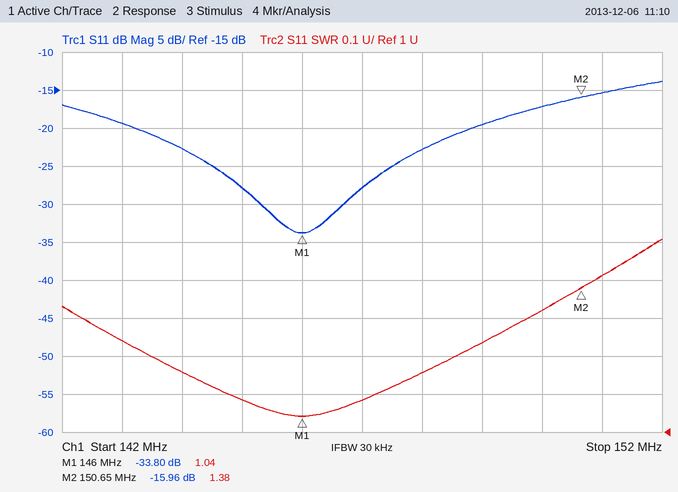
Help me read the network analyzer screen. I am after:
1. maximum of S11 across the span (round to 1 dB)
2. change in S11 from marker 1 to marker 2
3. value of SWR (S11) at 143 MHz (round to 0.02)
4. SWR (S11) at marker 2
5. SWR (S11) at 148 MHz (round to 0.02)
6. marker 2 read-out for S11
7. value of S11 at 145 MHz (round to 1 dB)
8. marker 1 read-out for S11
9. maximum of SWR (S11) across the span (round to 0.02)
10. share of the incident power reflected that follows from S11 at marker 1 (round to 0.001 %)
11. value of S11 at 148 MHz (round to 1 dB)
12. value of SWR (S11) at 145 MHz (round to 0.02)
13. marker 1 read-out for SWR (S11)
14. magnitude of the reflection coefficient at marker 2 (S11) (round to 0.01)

-14 dB
17.84 dB
1.24
1.38
1.16
-15.96 dB
-28 dB
-33.80 dB
1.50
0.042 %
-23 dB
1.08
1.04
0.16
